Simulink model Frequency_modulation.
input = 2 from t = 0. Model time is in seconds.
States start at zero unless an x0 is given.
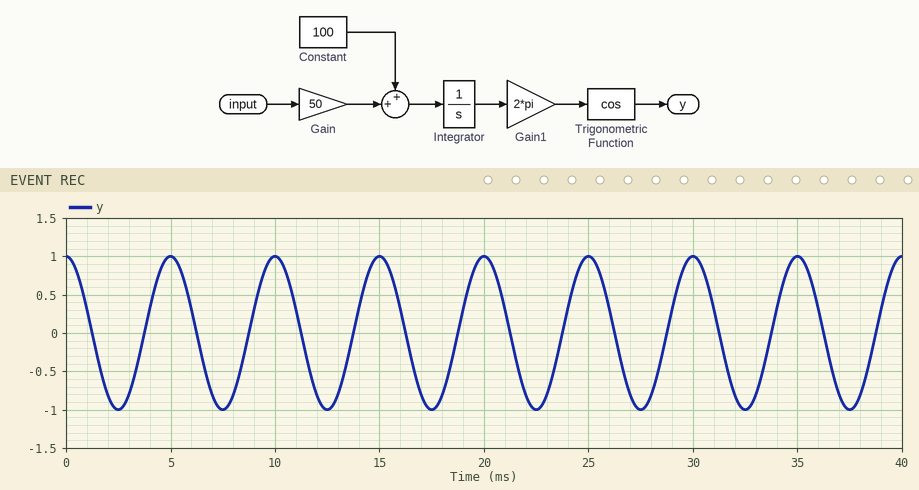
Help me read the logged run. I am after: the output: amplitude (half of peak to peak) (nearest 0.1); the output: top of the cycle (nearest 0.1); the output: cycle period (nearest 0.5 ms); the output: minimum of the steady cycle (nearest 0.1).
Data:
1.0
1.0
5.0 ms
-1.0
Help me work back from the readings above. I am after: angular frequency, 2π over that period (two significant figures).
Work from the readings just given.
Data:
1.3 rad/ms
